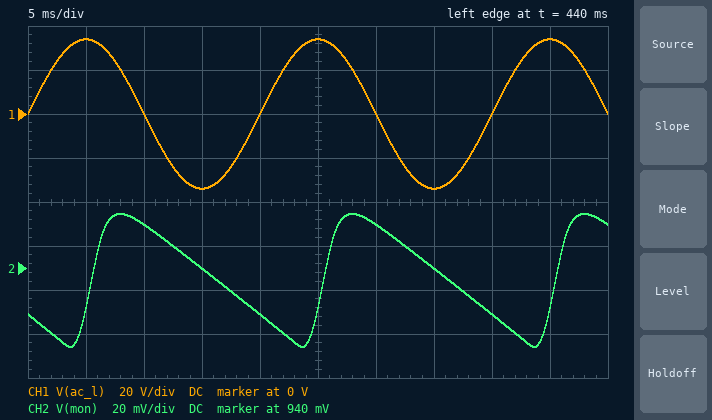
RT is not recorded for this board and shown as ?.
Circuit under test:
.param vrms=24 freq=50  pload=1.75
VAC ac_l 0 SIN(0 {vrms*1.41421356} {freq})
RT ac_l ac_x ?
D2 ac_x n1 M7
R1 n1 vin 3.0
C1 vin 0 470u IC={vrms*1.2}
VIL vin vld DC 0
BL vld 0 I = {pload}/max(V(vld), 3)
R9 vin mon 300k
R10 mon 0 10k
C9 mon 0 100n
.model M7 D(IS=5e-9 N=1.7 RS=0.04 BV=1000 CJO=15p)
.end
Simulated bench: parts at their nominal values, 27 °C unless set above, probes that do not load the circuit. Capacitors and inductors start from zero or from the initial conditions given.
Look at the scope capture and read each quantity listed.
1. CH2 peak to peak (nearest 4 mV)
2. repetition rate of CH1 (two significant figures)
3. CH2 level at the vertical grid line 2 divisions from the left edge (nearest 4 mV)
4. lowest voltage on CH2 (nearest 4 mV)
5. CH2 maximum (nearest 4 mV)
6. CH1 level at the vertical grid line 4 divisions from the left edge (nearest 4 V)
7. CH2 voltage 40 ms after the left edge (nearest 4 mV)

60 mV
50 Hz
960 mV
904 mV
964 mV
0 V
920 mV
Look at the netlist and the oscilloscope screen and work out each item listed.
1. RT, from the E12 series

3.9 Ω
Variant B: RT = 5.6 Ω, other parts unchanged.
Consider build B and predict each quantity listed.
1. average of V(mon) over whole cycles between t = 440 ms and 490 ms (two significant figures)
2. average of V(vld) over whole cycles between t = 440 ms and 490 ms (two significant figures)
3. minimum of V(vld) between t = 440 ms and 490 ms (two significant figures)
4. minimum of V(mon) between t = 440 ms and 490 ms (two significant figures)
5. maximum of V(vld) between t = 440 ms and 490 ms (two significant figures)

910 mV
28 V
27 V
880 mV
29 V
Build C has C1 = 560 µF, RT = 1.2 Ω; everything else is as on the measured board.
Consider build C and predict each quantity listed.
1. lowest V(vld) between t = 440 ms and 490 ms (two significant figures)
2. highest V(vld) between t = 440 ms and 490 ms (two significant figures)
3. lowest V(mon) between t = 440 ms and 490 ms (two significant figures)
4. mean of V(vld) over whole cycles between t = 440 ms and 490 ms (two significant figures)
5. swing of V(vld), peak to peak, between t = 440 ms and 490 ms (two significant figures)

29 V
31 V
950 mV
30 V
1.8 V
